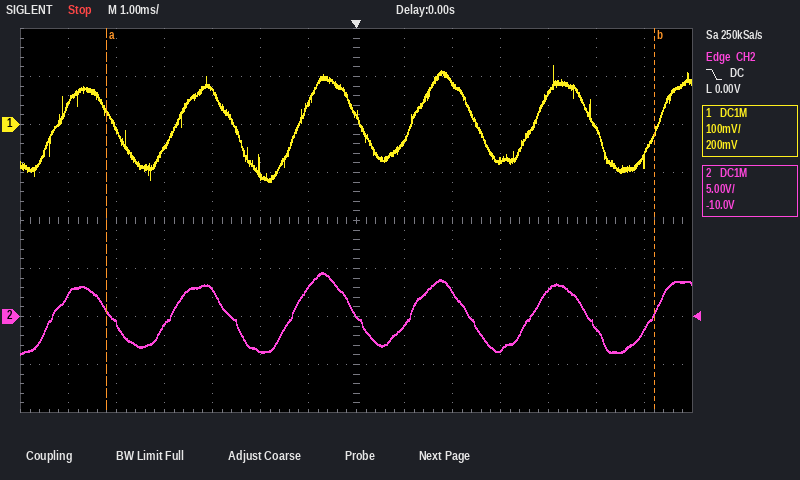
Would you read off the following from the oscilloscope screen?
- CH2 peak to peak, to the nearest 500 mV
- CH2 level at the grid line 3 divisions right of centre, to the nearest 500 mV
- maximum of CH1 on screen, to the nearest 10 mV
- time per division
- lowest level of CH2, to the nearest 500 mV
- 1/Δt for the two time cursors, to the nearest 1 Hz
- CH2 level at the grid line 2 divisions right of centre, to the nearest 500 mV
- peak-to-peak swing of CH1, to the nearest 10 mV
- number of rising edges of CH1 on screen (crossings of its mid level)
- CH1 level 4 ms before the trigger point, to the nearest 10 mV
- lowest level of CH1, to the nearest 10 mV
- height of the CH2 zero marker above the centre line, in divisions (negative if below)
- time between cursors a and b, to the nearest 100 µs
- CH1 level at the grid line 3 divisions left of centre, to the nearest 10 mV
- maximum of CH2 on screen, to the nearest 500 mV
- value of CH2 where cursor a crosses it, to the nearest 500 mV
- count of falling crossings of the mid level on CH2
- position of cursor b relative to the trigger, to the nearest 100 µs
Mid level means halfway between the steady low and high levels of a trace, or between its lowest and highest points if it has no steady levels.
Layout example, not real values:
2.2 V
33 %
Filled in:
8.5 V
-3.5 V
120 mV
1 ms
-4.0 V
88 Hz
2.5 V
240 mV
6
-50 mV
-120 mV
-2.0 div
11.4 ms
70 mV
4.5 V
500 mV
5
+6.2 ms
